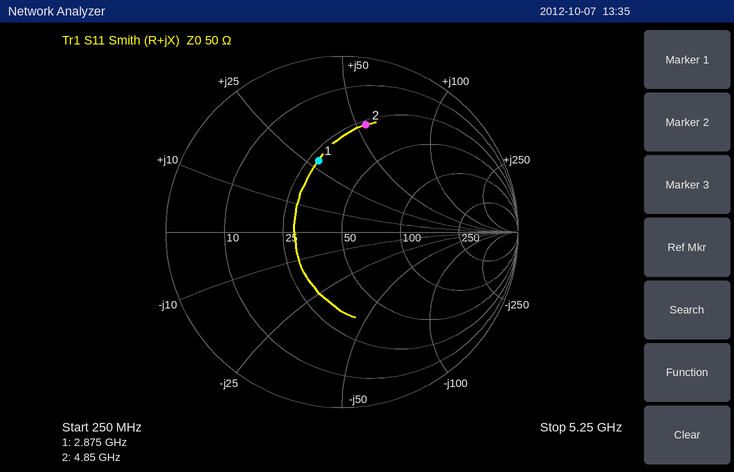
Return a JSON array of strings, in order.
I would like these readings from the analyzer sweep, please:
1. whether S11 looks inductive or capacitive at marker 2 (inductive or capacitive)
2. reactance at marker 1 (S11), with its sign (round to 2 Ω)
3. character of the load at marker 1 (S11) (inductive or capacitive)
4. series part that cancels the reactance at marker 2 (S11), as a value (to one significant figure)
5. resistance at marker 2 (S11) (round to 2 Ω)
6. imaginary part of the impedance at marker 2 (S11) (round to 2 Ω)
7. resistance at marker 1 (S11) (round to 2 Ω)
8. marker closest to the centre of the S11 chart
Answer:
["inductive", "+28 Ω", "inductive", "600 fF", "28 Ω", "+54 Ω", "28 Ω", "marker 1"]
